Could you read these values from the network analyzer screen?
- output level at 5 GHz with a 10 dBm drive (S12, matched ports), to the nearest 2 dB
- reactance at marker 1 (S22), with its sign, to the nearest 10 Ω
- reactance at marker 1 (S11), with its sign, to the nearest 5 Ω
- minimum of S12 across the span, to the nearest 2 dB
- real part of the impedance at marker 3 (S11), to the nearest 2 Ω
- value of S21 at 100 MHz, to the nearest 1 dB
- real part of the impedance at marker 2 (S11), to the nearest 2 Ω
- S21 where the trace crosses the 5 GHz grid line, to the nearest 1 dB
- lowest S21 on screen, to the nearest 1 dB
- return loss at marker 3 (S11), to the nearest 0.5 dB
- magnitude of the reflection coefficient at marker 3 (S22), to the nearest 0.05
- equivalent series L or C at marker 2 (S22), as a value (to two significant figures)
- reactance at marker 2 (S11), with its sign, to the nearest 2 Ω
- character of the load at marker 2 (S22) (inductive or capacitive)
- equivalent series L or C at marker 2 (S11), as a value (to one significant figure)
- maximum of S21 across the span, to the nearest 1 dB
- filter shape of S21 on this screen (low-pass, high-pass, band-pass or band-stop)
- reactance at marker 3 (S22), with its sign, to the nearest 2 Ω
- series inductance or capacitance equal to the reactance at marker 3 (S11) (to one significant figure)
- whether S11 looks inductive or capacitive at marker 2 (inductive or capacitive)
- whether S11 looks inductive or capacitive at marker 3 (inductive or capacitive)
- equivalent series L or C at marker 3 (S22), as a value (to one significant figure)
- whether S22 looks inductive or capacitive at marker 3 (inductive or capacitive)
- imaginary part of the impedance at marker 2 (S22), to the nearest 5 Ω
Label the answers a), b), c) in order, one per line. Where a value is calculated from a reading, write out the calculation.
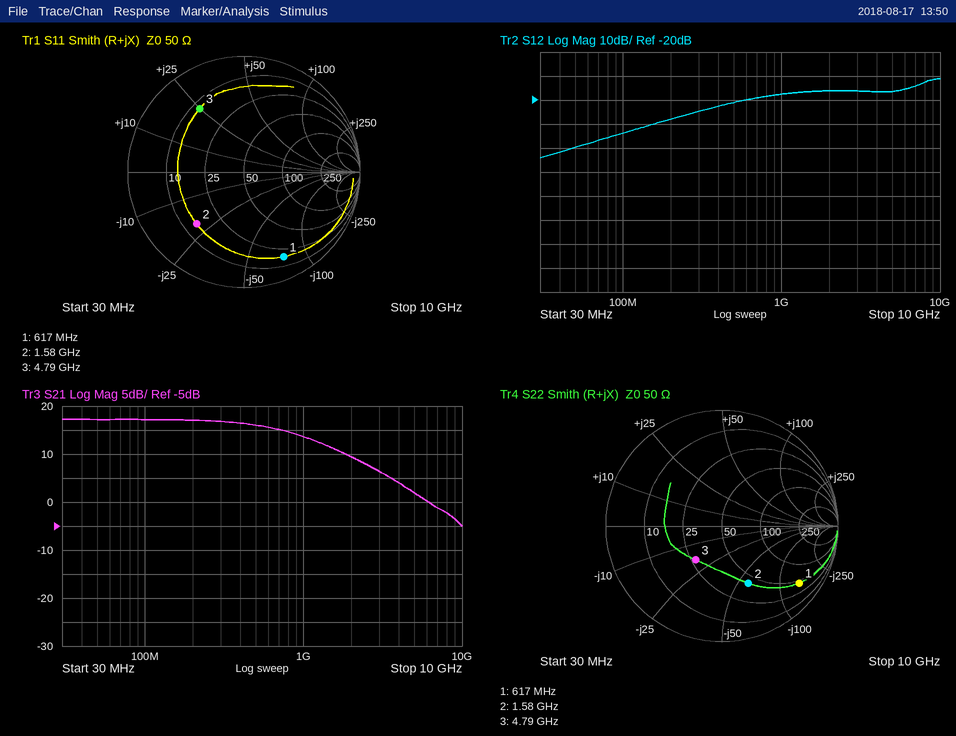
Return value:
a) 10 dBm + (-16 dB) = -6 dBm
b) -140 Ω
c) -75 Ω
d) -44 dB
e) 12 Ω
f) 17 dB
g) 14 Ω
h) 2 dB
i) -5 dB
j) 3.5 dB
k) 0.35
l) C = 1/(2π × 1.58 GHz × 60 Ω) ≈ 1.7 pF
m) -20 Ω
n) capacitive
o) C = 1/(2π × 1.58 GHz × 20 Ω) ≈ 5 pF
p) 17 dB
q) low-pass
r) -18 Ω
s) L = 24 Ω/(2π × 4.79 GHz) ≈ 797 pH, so 800 pH to one significant figure
t) capacitive
u) inductive
v) C = 1/(2π × 4.79 GHz × 18 Ω) ≈ 2 pF
w) capacitive
x) -60 Ω
